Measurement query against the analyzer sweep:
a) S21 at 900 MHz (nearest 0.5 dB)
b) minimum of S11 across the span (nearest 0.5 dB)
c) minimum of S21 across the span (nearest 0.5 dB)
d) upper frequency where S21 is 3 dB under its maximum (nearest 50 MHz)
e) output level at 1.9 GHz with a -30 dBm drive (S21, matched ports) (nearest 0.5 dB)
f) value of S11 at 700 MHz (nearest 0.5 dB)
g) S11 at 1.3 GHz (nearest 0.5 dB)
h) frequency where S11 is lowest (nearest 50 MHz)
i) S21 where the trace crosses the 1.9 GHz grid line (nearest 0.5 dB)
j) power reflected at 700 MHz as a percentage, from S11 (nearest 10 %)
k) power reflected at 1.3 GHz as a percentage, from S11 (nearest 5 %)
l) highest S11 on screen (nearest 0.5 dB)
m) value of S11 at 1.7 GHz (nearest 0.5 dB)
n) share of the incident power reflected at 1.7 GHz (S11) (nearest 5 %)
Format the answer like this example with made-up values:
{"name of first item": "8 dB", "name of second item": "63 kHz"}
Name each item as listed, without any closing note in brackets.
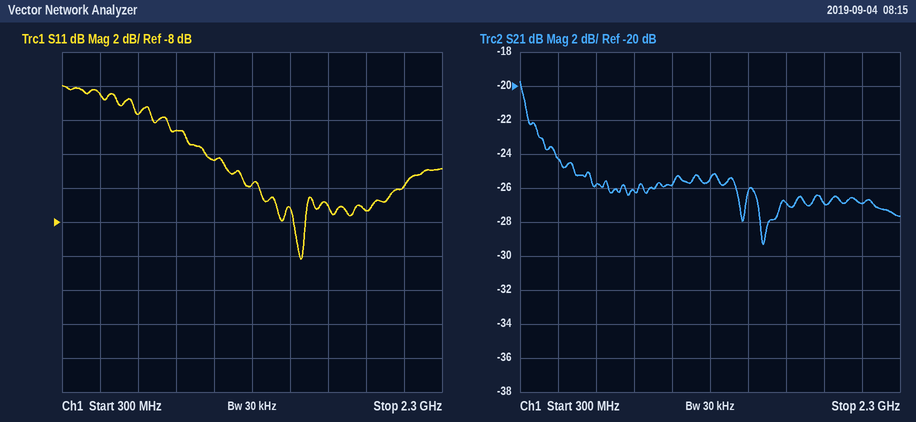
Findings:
{"S21 at 900 MHz": "-26.0 dB", "minimum of S11 across the span": "-10.0 dB", "minimum of S21 across the span": "-29.5 dB", "upper frequency where S21 is 3 dB under its maximum": "400 MHz", "output level at 1.9 GHz with a -30 dBm drive (S21, matched ports)": "-57.0 dBm", "value of S11 at 700 MHz": "-1.5 dB", "S11 at 1.3 GHz": "-6.0 dB", "frequency where S11 is lowest": "1.55 GHz", "S21 where the trace crosses the 1.9 GHz grid line": "-27.0 dB", "power reflected at 700 MHz as a percentage, from S11": "70 %", "power reflected at 1.3 GHz as a percentage, from S11": "25 %", "highest S11 on screen": "0.0 dB", "value of S11 at 1.7 GHz": "-7.0 dB", "share of the incident power reflected at 1.7 GHz (S11)": "20 %"}
